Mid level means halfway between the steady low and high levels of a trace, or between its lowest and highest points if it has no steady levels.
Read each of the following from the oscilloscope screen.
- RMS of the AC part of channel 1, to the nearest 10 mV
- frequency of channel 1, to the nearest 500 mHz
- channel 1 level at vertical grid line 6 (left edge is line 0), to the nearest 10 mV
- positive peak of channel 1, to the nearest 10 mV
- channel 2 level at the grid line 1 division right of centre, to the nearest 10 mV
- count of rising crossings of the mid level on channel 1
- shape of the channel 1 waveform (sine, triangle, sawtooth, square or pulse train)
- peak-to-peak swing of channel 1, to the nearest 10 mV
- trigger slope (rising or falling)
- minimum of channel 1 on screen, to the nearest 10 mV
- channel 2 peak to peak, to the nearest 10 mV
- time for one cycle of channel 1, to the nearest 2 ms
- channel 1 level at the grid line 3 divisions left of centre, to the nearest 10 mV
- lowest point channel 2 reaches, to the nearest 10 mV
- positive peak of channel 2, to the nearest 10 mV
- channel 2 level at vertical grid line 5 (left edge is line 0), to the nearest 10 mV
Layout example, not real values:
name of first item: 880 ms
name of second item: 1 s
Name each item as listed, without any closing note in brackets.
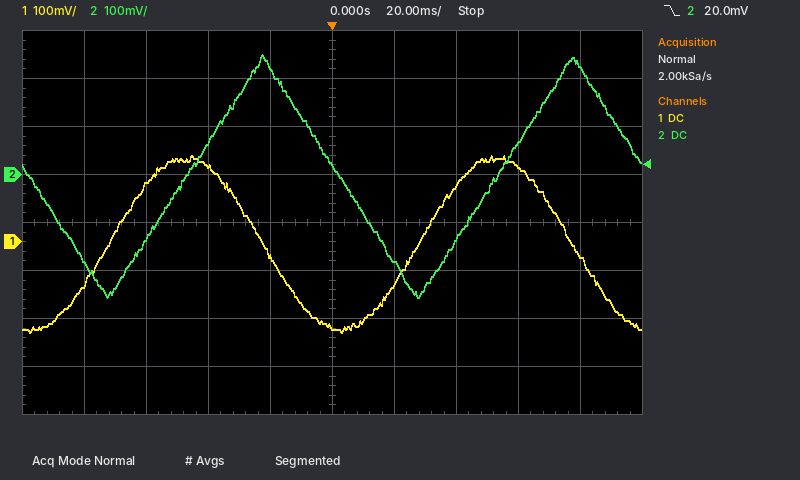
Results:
RMS of the AC part of channel 1, to the nearest 10 mV: 130 mV
frequency of channel 1, to the nearest 500 mHz: 10.0 Hz
channel 1 level at vertical grid line 6 (left edge is line 0), to the nearest 10 mV: -90 mV
positive peak of channel 1, to the nearest 10 mV: 180 mV
channel 2 level at the grid line 1 division right of centre, to the nearest 10 mV: -180 mV
count of rising crossings of the mid level on channel 1: 2
shape of the channel 1 waveform: sine
peak-to-peak swing of channel 1, to the nearest 10 mV: 370 mV
trigger slope: falling
minimum of channel 1 on screen, to the nearest 10 mV: -190 mV
channel 2 peak to peak, to the nearest 10 mV: 510 mV
time for one cycle of channel 1, to the nearest 2 ms: 100 ms
channel 1 level at the grid line 3 divisions left of centre, to the nearest 10 mV: 120 mV
lowest point channel 2 reaches, to the nearest 10 mV: -260 mV
positive peak of channel 2, to the nearest 10 mV: 250 mV
channel 2 level at vertical grid line 5 (left edge is line 0), to the nearest 10 mV: 20 mV
